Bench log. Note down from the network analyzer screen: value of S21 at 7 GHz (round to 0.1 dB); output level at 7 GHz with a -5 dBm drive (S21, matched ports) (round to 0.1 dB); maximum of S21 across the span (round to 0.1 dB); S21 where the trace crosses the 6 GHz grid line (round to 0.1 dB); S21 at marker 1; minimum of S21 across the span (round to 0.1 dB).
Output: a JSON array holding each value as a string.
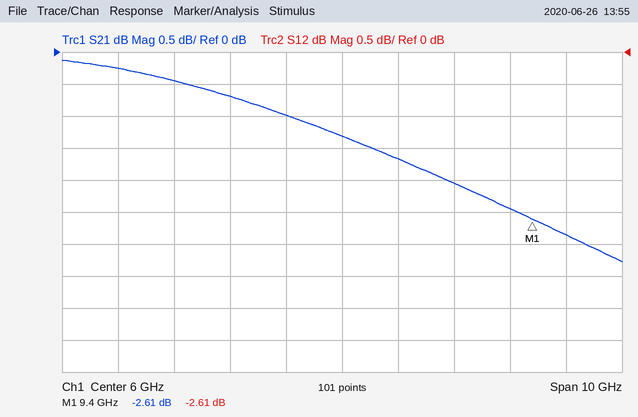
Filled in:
["-1.7 dB", "-6.7 dBm", "-0.1 dB", "-1.3 dB", "-2.61 dB", "-3.3 dB"]
